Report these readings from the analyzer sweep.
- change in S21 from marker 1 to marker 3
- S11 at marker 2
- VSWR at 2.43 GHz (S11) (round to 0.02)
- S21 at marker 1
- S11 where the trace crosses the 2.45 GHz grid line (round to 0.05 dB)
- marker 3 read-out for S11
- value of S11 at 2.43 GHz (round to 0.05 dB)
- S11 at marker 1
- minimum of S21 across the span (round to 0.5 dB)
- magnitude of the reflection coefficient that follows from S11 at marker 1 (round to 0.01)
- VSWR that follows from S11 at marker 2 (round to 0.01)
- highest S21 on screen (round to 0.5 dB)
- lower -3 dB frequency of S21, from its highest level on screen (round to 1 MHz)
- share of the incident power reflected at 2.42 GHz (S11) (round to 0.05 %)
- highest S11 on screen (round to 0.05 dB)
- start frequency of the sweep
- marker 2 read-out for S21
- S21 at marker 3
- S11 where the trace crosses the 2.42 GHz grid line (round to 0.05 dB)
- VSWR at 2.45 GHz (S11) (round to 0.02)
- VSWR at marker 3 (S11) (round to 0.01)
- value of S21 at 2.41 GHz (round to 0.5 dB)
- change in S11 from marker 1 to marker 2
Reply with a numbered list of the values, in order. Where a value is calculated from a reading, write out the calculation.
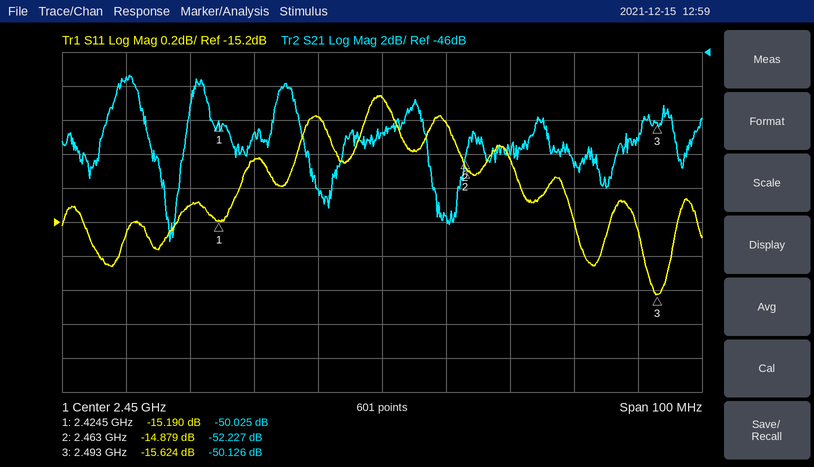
1. -50.126 − (-50.025) = -0.101 dB
2. -14.879 dB
3. |Γ| = 10^(-14.85/20) = 0.1809; VSWR = (1 + 0.1809)/(1 − 0.1809) ≈ 1.44
4. -50.025 dB
5. -14.45 dB
6. -15.624 dB
7. -14.85 dB
8. -15.190 dB
9. -57.0 dB
10. 10^(-15.19/20) ≈ 0.17
11. (1 + 0.1803)/(1 − 0.1803) ≈ 1.44
12. -47.5 dB
13. 2.407 GHz
14. 10^(-15.1/10) ≈ 3.09 %, so 3.10 % to the nearest 0.05 %
15. -14.45 dB
16. 2.4 GHz
17. -52.227 dB
18. -50.126 dB
19. -15.10 dB
20. |Γ| = 10^(-14.45/20) = 0.1895; VSWR = (1 + 0.1895)/(1 − 0.1895) ≈ 1.47, so 1.46 to the nearest 0.02
21. (1 + 0.1655)/(1 − 0.1655) ≈ 1.40
22. -47.5 dB
23. -14.879 − (-15.19) = 0.311 dB
